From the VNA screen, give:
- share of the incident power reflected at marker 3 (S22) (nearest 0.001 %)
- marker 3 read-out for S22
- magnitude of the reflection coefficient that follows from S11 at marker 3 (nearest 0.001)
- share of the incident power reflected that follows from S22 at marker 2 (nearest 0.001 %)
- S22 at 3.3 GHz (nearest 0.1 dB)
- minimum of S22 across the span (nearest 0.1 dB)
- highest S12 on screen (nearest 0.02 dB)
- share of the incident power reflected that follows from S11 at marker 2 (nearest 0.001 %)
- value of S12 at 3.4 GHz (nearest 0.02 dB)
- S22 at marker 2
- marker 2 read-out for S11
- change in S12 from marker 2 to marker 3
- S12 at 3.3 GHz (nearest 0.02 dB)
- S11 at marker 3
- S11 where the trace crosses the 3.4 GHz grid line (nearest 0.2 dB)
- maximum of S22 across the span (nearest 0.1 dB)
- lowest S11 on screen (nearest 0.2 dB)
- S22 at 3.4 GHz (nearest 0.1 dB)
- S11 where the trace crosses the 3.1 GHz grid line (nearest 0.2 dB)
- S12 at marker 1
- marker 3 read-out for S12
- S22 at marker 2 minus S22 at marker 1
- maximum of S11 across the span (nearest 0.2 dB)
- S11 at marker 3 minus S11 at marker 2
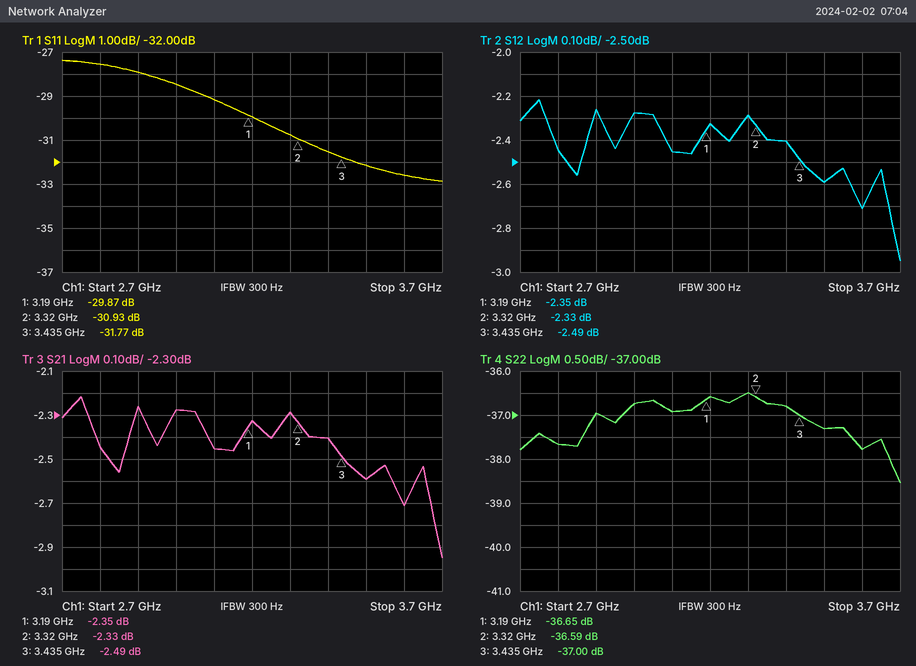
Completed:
0.020 %
-37.00 dB
0.026
0.022 %
-36.5 dB
-38.5 dB
-2.22 dB
0.081 %
-2.40 dB
-36.59 dB
-30.93 dB
-0.16 dB
-2.28 dB
-31.77 dB
-31.6 dB
-36.5 dB
-32.8 dB
-36.8 dB
-29.2 dB
-2.35 dB
-2.49 dB
0.06 dB
-27.4 dB
-0.84 dB
